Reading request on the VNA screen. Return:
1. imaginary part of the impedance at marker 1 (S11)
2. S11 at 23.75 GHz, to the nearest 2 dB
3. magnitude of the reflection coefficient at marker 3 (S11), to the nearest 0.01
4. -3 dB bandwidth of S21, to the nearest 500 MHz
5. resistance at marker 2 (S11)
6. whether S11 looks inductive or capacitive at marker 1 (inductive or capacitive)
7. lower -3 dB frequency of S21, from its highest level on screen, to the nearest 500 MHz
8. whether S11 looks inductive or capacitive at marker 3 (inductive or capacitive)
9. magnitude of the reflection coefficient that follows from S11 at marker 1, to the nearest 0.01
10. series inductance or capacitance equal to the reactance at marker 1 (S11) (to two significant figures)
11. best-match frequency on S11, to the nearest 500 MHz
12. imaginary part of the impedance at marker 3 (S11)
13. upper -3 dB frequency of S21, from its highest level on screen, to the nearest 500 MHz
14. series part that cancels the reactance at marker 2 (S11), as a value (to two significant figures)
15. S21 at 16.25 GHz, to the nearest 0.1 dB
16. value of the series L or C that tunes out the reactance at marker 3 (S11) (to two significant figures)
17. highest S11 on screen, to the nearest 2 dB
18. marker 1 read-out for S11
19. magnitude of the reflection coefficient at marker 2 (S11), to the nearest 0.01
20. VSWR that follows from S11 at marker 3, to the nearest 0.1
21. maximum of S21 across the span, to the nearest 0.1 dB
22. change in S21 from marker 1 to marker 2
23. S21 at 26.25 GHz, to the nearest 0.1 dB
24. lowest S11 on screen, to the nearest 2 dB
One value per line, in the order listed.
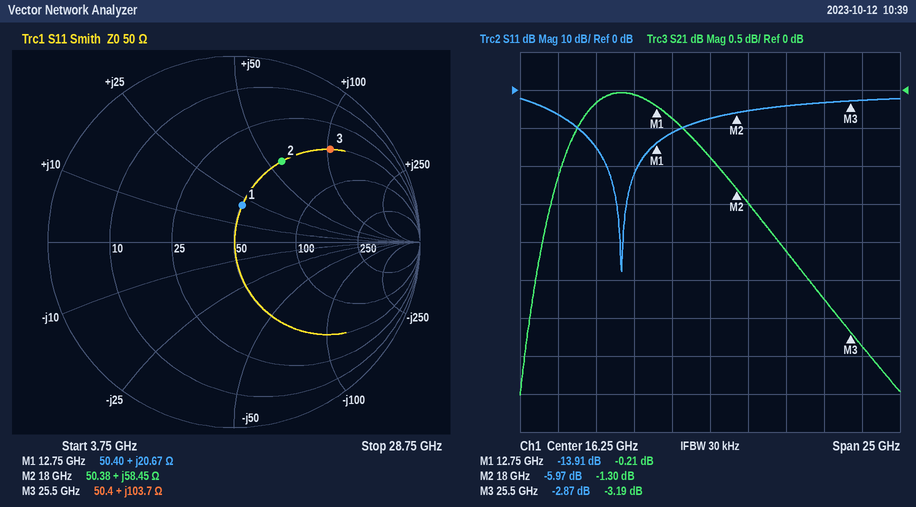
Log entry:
+20.67 Ω
-4 dB
0.72
20.5 GHz
50.38 Ω
inductive
4.5 GHz
inductive
0.20
260 pH
10.5 GHz
+103.7 Ω
25.0 GHz
150 fF
-0.9 dB
60 fF
-2 dB
-13.91 dB
0.50
6.1
0.0 dB
-1.09 dB
-3.4 dB
-48 dB
